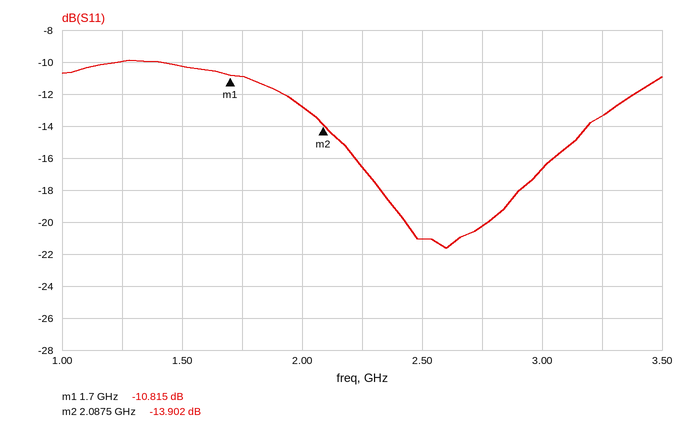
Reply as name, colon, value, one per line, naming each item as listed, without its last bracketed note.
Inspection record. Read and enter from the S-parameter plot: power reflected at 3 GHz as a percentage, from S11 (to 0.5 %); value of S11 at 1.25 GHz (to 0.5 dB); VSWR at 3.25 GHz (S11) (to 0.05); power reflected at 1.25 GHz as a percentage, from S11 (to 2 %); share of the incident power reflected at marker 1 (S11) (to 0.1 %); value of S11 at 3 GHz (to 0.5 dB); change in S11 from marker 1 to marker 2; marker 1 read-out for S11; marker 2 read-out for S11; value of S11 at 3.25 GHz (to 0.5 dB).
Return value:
power reflected at 3 GHz as a percentage, from S11: 2.0 %
value of S11 at 1.25 GHz: -10.0 dB
VSWR at 3.25 GHz (S11): 1.55
power reflected at 1.25 GHz as a percentage, from S11: 10 %
share of the incident power reflected at marker 1 (S11): 8.3 %
value of S11 at 3 GHz: -16.5 dB
change in S11 from marker 1 to marker 2: -3.087 dB
marker 1 read-out for S11: -10.815 dB
marker 2 read-out for S11: -13.902 dB
value of S11 at 3.25 GHz: -13.5 dB
